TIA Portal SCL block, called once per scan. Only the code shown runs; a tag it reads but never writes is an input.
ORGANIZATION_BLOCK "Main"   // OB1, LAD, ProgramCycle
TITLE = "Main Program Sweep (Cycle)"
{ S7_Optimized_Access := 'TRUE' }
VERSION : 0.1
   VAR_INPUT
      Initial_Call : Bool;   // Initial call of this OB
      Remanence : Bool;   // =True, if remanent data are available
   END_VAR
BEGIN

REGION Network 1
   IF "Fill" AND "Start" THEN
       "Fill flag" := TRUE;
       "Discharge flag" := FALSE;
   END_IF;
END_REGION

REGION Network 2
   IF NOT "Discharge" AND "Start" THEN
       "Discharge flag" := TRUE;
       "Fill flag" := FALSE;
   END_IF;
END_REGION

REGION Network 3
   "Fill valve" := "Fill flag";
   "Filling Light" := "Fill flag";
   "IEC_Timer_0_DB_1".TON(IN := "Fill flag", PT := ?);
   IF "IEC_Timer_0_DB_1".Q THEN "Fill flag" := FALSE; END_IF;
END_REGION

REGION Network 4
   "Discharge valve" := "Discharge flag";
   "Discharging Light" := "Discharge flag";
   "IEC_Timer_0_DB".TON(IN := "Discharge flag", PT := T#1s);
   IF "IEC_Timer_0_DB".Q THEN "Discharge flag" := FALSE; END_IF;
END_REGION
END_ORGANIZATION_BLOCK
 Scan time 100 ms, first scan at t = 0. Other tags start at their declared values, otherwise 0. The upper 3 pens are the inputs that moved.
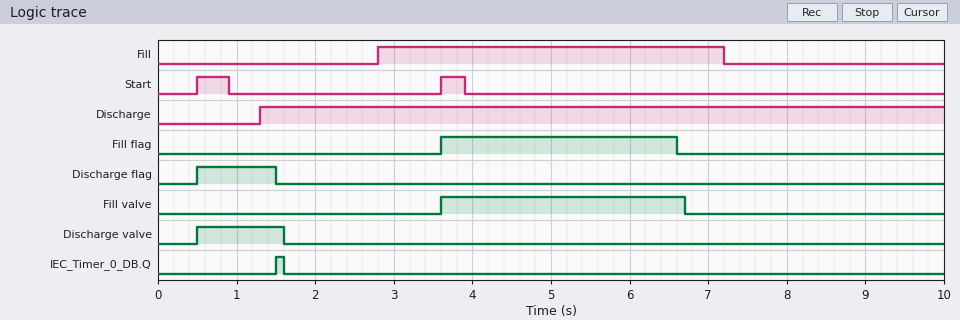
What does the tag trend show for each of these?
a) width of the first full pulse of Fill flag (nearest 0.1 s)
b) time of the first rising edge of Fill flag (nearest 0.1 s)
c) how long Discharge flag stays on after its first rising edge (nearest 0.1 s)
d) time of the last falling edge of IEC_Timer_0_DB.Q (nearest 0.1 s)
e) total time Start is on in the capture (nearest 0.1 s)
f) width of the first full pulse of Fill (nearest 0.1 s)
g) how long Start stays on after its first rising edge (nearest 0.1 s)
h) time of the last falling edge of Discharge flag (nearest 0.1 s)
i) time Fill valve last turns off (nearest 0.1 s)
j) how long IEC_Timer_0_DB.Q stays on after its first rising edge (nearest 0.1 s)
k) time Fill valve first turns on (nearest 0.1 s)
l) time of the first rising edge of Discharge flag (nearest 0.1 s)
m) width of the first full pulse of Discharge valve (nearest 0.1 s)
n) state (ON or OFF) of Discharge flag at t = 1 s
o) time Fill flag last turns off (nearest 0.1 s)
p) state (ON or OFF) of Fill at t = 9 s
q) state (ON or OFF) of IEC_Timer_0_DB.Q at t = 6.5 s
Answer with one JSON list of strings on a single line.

["3.0 s", "3.6 s", "1.0 s", "1.6 s", "0.7 s", "4.4 s", "0.4 s", "1.5 s", "6.7 s", "0.1 s", "3.6 s", "0.5 s", "1.1 s", "ON", "6.6 s", "OFF", "OFF"]
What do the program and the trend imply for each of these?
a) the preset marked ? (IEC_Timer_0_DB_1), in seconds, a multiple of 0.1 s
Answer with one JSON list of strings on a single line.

["3.0 s"]
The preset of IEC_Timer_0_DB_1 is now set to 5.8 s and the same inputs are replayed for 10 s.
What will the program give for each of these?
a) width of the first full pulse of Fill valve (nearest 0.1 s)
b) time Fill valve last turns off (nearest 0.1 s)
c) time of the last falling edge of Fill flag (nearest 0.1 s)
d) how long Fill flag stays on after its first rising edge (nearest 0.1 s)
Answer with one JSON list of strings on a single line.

["5.9 s", "9.5 s", "9.4 s", "5.8 s"]
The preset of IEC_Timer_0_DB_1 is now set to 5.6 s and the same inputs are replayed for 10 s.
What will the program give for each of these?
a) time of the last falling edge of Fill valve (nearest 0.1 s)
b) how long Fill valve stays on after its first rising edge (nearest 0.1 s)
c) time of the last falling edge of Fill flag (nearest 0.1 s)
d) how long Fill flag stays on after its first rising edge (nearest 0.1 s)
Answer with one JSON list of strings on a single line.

["9.3 s", "5.7 s", "9.2 s", "5.6 s"]
